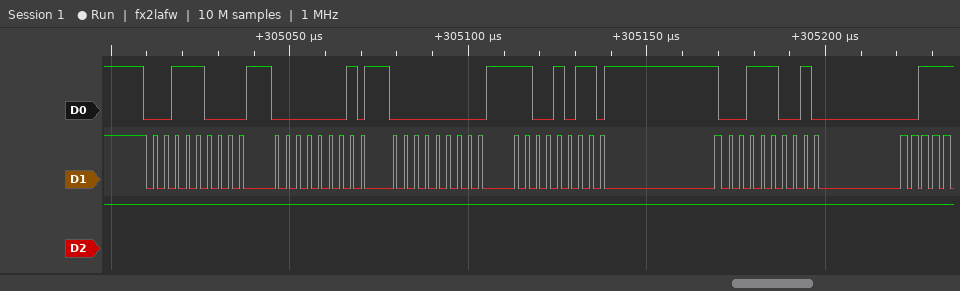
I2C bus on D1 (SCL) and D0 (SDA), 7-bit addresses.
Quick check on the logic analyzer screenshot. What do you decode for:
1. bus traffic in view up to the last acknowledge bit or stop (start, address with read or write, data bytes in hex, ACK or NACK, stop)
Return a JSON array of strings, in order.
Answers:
["start, address 1C write ACK, 01 ACK, 00 ACK, CB ACK, repeated start, address 1C read ACK"]
